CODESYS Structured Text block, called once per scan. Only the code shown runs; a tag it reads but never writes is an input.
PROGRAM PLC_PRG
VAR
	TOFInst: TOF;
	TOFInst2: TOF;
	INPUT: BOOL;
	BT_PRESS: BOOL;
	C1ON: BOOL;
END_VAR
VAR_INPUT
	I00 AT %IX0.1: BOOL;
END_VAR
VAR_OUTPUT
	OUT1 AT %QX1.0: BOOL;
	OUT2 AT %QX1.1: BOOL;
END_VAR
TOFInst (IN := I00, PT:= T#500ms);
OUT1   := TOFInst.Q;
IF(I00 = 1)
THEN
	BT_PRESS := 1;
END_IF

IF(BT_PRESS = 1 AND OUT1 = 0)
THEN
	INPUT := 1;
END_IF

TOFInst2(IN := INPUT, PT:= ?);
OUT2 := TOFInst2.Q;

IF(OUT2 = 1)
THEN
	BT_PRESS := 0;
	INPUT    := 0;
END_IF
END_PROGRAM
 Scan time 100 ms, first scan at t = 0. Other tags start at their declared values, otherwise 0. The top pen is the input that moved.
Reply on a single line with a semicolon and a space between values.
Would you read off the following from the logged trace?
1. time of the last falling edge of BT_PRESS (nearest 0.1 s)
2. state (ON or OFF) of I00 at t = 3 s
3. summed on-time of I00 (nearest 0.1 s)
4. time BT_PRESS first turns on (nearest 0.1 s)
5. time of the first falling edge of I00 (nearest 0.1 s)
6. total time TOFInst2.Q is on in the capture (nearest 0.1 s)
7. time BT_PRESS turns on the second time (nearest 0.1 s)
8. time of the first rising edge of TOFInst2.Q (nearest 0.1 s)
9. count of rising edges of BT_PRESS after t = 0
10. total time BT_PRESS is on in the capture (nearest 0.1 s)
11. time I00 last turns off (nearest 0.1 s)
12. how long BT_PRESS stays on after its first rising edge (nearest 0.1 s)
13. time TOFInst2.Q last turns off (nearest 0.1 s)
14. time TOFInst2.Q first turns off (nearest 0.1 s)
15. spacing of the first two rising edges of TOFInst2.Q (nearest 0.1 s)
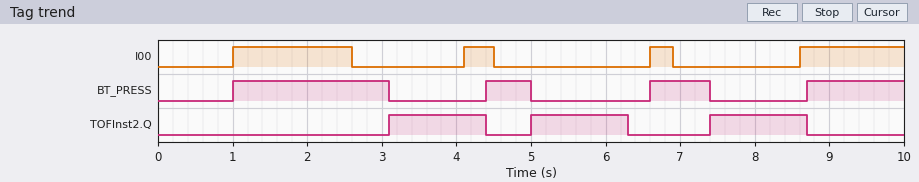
7.4 s; OFF; 3.7 s; 1.0 s; 2.6 s; 3.9 s; 4.4 s; 3.1 s; 4; 4.8 s; 6.9 s; 2.1 s; 8.7 s; 4.4 s; 1.9 s
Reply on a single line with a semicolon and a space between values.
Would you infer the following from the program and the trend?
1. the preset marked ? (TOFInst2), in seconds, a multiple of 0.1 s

1.2 s
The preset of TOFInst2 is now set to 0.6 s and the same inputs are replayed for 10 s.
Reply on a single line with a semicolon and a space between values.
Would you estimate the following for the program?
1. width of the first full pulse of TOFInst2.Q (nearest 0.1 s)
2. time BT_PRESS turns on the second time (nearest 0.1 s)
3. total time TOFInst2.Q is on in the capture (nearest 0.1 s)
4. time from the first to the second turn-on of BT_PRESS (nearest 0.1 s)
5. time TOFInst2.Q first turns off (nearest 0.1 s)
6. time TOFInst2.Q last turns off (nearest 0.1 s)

0.7 s; 4.1 s; 2.1 s; 3.1 s; 3.8 s; 8.1 s
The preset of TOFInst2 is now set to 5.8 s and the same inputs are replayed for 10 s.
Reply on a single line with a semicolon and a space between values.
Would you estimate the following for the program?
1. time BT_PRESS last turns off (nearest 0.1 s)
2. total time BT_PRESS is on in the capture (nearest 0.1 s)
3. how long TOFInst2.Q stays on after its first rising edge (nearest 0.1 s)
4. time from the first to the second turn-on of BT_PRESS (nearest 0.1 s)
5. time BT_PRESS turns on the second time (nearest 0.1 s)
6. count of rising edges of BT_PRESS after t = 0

3.1 s; 3.1 s; 5.9 s; 8.0 s; 9.0 s; 2
